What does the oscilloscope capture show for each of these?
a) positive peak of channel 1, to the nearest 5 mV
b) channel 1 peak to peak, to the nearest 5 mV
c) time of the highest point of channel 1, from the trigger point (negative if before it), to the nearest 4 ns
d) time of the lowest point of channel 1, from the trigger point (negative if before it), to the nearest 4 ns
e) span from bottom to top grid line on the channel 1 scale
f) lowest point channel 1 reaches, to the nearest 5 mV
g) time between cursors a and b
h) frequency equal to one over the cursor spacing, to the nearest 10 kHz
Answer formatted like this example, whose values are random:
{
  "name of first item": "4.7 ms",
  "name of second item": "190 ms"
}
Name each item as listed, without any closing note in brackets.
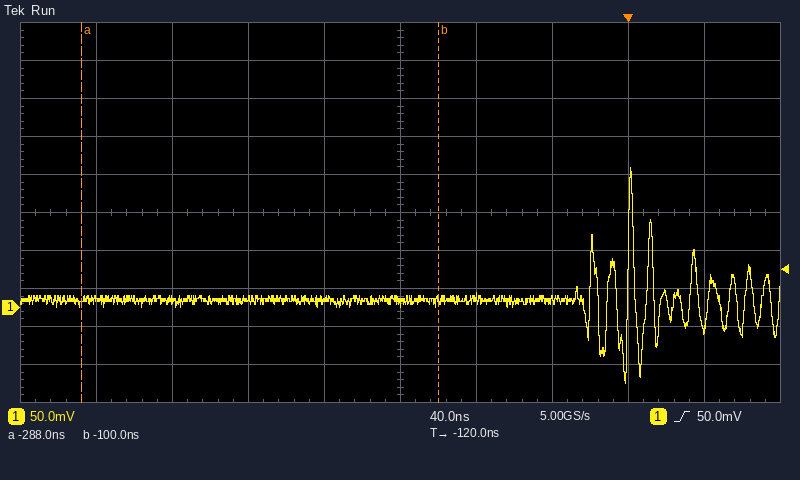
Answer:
{
  "positive peak of channel 1, to the nearest 5 mV": "185 mV",
  "channel 1 peak to peak, to the nearest 5 mV": "285 mV",
  "time of the highest point of channel 1, from the trigger point (negative if before it), to the nearest 4 ns": "0 ns",
  "time of the lowest point of channel 1, from the trigger point (negative if before it), to the nearest 4 ns": "0 ns",
  "span from bottom to top grid line on the channel 1 scale": "500 mV",
  "lowest point channel 1 reaches, to the nearest 5 mV": "-100 mV",
  "time between cursors a and b": "188 ns",
  "frequency equal to one over the cursor spacing, to the nearest 10 kHz": "5.32 MHz"
}
